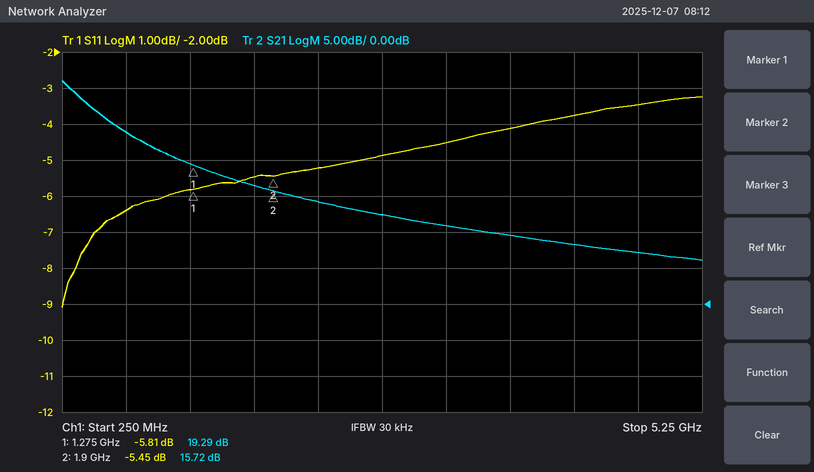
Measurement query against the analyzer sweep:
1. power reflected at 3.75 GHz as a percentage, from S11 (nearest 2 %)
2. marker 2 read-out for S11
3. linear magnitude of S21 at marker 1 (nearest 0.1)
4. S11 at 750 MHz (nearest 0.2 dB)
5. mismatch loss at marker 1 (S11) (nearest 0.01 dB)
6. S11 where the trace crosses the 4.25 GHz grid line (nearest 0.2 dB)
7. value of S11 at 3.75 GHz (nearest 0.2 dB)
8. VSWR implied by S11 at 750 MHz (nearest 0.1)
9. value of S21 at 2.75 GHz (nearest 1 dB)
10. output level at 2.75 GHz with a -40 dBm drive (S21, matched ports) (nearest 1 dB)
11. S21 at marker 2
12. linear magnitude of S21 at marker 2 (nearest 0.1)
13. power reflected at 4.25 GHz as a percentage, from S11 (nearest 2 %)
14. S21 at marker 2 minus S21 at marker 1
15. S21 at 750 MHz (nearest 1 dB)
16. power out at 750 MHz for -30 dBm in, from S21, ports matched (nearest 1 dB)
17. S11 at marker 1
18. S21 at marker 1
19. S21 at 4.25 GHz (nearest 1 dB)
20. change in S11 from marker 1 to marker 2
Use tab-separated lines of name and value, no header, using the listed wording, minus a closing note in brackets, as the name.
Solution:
power reflected at 3.75 GHz as a percentage, from S11	38 %
marker 2 read-out for S11	-5.45 dB
linear magnitude of S21 at marker 1	9.2
S11 at 750 MHz	-6.4 dB
mismatch loss at marker 1 (S11)	1.32 dB
S11 where the trace crosses the 4.25 GHz grid line	-3.8 dB
value of S11 at 3.75 GHz	-4.2 dB
VSWR implied by S11 at 750 MHz	2.8
value of S21 at 2.75 GHz	12 dB
output level at 2.75 GHz with a -40 dBm drive (S21, matched ports)	-28 dBm
S21 at marker 2	15.72 dB
linear magnitude of S21 at marker 2	6.1
power reflected at 4.25 GHz as a percentage, from S11	42 %
S21 at marker 2 minus S21 at marker 1	-3.57 dB
S21 at 750 MHz	24 dB
power out at 750 MHz for -30 dBm in, from S21, ports matched	-6 dBm
S11 at marker 1	-5.81 dB
S21 at marker 1	19.29 dB
S21 at 4.25 GHz	8 dB
change in S11 from marker 1 to marker 2	0.36 dB
